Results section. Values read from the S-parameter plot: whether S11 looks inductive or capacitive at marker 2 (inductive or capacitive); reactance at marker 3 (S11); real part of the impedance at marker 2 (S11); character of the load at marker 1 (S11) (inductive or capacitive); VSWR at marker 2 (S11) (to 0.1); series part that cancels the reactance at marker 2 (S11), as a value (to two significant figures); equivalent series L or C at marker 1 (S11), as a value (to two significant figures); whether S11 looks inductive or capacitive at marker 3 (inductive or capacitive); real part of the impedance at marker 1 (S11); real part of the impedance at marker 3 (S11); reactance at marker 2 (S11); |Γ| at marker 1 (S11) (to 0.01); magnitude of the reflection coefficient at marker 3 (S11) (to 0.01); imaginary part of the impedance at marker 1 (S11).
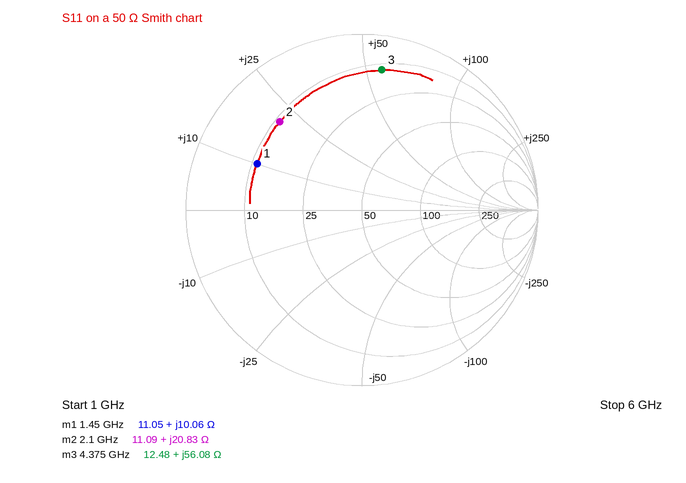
inductive
+56.08 Ω
11.09 Ω
inductive
5.3
3.6 pF
1.1 nH
inductive
11.05 Ω
12.48 Ω
+20.83 Ω
0.65
0.80
+10.06 Ω
